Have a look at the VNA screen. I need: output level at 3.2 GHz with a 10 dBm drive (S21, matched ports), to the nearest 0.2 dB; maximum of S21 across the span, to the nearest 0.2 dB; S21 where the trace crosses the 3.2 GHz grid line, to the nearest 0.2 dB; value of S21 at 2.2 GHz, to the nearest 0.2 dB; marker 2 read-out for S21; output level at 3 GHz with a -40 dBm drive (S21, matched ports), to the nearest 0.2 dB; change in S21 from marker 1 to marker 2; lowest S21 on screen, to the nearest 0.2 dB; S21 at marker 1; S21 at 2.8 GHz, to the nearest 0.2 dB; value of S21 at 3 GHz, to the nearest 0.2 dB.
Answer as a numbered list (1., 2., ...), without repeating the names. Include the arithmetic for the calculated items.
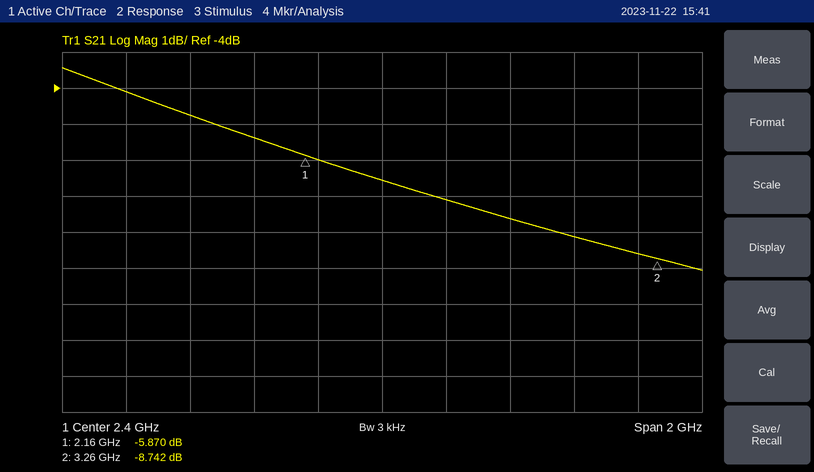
1. 10 dBm + (-8.6 dB) = 1.4 dBm
2. -3.4 dB
3. -8.6 dB
4. -6.0 dB
5. -8.742 dB
6. -40 dBm + (-8.2 dB) = -48.2 dBm
7. -8.742 − (-5.87) = -2.872 dB
8. -9.0 dB
9. -5.870 dB
10. -7.6 dB
11. -8.2 dB
